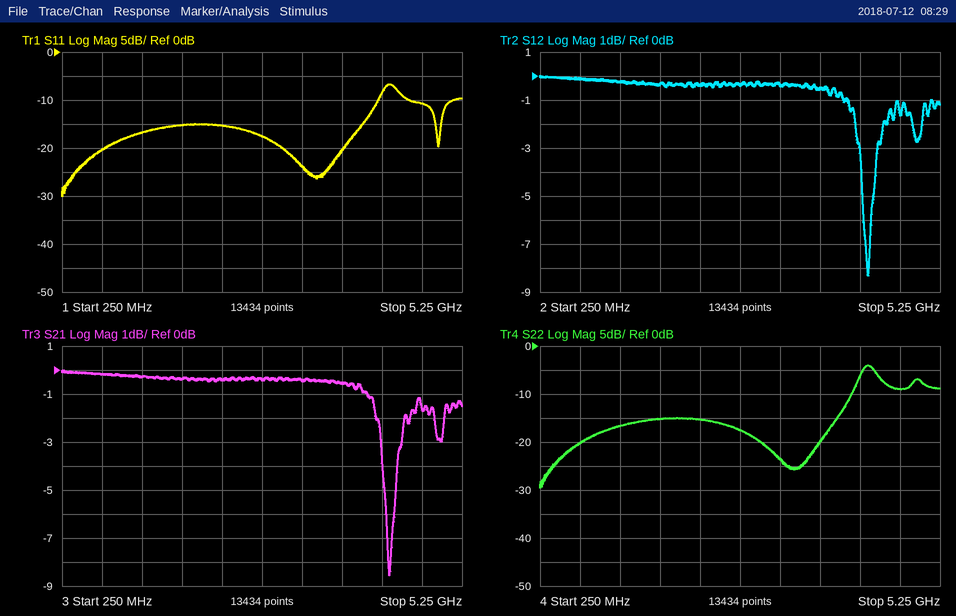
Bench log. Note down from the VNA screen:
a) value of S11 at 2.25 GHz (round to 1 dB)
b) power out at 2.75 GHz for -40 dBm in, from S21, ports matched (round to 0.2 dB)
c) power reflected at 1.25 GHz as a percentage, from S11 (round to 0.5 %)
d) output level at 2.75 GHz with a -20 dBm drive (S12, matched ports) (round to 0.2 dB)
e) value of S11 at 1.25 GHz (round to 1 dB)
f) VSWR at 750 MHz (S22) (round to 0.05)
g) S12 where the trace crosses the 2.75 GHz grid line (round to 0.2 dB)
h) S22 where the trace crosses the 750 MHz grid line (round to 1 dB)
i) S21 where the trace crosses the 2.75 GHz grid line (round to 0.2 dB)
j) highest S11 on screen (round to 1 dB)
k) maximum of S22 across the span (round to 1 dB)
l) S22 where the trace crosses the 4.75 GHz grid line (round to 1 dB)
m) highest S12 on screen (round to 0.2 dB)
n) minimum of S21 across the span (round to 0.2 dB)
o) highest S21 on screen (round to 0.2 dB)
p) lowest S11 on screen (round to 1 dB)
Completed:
-15 dB
-40.4 dBm
2.0 %
-20.4 dBm
-17 dB
1.20
-0.4 dB
-20 dB
-0.4 dB
-7 dB
-4 dB
-9 dB
0.0 dB
-8.6 dB
0.0 dB
-30 dB
